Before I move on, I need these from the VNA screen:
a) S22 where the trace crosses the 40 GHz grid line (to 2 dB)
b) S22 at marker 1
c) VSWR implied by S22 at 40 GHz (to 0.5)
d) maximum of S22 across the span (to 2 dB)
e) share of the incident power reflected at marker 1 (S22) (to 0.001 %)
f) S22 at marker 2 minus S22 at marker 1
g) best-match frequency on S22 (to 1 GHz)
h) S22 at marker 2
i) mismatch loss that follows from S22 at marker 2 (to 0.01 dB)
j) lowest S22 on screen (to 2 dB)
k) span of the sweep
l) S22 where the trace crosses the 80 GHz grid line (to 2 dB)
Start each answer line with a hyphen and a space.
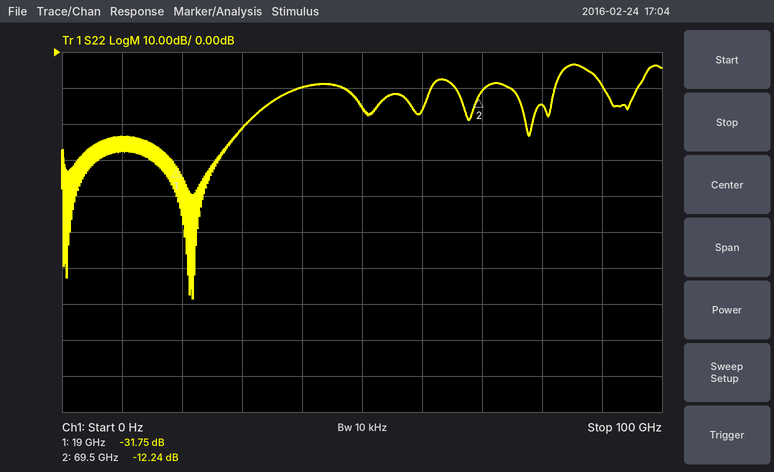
- -10 dB
- -31.75 dB
- 2.0
- -4 dB
- 0.067 %
- 19.51 dB
- 22 GHz
- -12.24 dB
- 0.27 dB
- -68 dB
- 100 GHz
- -14 dB
